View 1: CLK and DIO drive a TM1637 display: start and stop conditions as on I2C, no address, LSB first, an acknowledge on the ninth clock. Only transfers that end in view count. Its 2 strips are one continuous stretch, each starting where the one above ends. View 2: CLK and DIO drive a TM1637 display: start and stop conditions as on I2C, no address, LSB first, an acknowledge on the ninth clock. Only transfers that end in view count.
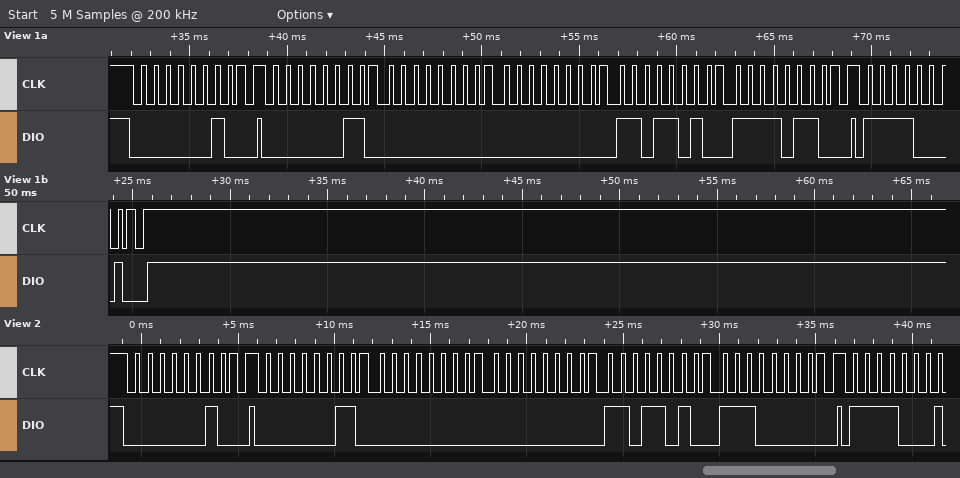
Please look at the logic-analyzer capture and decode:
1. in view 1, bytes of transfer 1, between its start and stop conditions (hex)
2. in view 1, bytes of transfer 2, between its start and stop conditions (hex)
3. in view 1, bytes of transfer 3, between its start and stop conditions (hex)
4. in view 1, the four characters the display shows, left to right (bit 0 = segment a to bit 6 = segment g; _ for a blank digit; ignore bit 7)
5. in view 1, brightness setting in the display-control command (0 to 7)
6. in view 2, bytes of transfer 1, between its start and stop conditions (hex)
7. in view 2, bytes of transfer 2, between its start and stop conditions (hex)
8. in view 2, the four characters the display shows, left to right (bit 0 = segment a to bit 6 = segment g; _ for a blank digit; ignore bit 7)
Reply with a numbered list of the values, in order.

1. 40
2. C0 00 00 5B 6F
3. 8F
4. __29
5. 7
6. 40
7. C0 00 00 5B 07
8. __27
